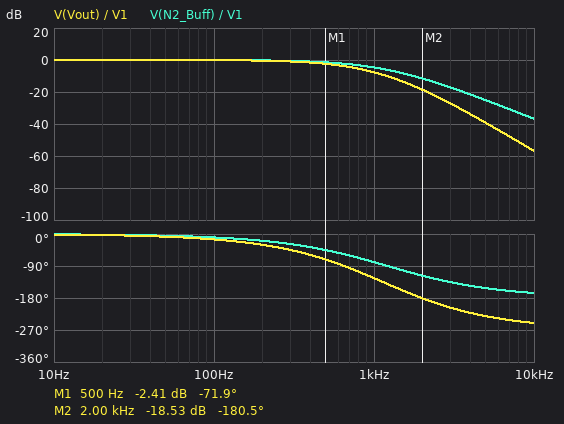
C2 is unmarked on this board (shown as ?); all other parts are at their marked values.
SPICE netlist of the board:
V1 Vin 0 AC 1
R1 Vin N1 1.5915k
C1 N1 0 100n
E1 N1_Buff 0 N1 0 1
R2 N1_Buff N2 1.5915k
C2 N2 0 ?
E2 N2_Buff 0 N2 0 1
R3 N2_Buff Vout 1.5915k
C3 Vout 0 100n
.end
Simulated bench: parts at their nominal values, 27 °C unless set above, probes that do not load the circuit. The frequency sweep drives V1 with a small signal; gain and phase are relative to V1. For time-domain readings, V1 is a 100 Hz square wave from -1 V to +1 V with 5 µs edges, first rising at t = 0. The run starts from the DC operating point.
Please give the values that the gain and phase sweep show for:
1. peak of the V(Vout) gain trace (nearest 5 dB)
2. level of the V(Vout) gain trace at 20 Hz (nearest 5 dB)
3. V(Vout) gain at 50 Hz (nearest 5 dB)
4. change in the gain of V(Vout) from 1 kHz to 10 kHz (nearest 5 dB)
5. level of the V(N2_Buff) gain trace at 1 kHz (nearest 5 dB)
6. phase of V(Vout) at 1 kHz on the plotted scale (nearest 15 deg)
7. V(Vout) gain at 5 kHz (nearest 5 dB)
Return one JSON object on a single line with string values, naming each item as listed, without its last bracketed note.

{"peak of the V(Vout) gain trace": "0 dB", "level of the V(Vout) gain trace at 20 Hz": "0 dB", "V(Vout) gain at 50 Hz": "0 dB", "change in the gain of V(Vout) from 1 kHz to 10 kHz": "-50 dB", "level of the V(N2_Buff) gain trace at 1 kHz": "-5 dB", "phase of V(Vout) at 1 kHz on the plotted scale": "-120 deg", "V(Vout) gain at 5 kHz": "-40 dB"}
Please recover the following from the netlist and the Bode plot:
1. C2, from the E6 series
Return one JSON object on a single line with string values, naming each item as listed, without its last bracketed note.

{"C2, from the E6 series": "68 nF"}
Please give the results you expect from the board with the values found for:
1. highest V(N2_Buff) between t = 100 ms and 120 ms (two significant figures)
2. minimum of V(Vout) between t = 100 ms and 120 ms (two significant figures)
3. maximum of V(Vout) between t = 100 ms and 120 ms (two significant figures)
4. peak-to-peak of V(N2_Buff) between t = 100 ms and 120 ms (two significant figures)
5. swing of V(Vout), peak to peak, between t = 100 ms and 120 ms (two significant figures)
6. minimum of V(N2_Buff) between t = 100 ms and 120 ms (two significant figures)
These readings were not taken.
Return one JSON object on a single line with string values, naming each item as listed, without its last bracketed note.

{"highest V(N2_Buff) between t = 100 ms and 120 ms": "1.0 V", "minimum of V(Vout) between t = 100 ms and 120 ms": "-1.0 V", "maximum of V(Vout) between t = 100 ms and 120 ms": "1.0 V", "peak-to-peak of V(N2_Buff) between t = 100 ms and 120 ms": "2.0 V", "swing of V(Vout), peak to peak, between t = 100 ms and 120 ms": "2.0 V", "minimum of V(N2_Buff) between t = 100 ms and 120 ms": "-1.0 V"}
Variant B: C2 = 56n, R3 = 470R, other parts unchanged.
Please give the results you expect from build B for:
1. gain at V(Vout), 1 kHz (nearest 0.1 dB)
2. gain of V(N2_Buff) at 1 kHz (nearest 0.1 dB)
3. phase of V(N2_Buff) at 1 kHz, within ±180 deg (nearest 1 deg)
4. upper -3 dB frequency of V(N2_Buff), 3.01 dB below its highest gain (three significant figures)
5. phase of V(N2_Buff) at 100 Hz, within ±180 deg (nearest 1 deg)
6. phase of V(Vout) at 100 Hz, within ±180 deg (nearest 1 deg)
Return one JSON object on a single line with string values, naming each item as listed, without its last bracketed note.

{"gain at V(Vout), 1 kHz": "-4.6 dB", "gain of V(N2_Buff) at 1 kHz": "-4.2 dB", "phase of V(N2_Buff) at 1 kHz, within ±180 deg": "-74 deg", "upper -3 dB frequency of V(N2_Buff), 3.01 dB below its highest gain": "811 Hz", "phase of V(N2_Buff) at 100 Hz, within ±180 deg": "-9 deg", "phase of V(Vout) at 100 Hz, within ±180 deg": "-11 deg"}
